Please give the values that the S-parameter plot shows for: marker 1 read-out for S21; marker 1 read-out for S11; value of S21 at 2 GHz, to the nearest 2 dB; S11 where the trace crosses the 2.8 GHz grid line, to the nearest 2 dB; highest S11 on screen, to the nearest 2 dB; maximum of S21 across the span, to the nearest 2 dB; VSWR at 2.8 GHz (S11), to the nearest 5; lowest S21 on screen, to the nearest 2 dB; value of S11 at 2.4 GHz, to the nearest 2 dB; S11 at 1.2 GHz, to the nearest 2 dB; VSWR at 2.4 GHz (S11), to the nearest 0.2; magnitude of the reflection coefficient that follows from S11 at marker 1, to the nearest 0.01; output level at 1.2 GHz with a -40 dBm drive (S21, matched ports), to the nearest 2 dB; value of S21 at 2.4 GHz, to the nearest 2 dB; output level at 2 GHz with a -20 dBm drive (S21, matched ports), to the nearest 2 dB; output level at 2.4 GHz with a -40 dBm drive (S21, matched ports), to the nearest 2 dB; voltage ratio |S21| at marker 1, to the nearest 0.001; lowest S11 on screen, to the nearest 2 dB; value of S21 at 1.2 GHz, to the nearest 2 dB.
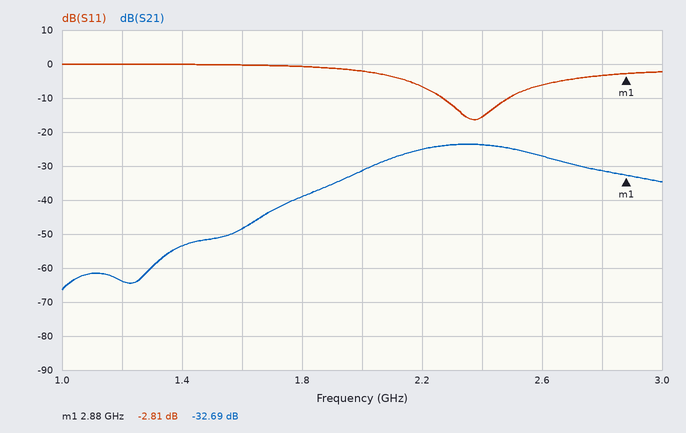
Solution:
-32.69 dB
-2.81 dB
-32 dB
-4 dB
0 dB
-24 dB
5
-66 dB
-16 dB
0 dB
1.4
0.72
-104 dBm
-24 dB
-52 dBm
-64 dBm
0.023
-16 dB
-64 dB
